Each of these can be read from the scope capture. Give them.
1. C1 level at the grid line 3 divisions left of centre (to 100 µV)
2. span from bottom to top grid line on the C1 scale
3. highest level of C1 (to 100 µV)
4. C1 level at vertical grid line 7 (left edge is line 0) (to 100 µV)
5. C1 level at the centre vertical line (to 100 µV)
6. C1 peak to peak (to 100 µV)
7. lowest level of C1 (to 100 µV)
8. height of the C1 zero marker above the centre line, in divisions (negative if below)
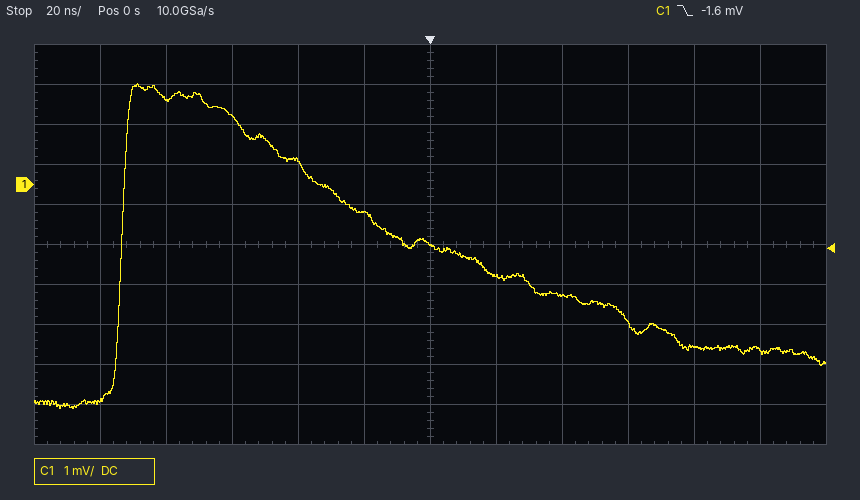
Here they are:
1.7 mV
10 mV
2.5 mV
-2.3 mV
-1.5 mV
8.1 mV
-5.6 mV
+1.5 div
